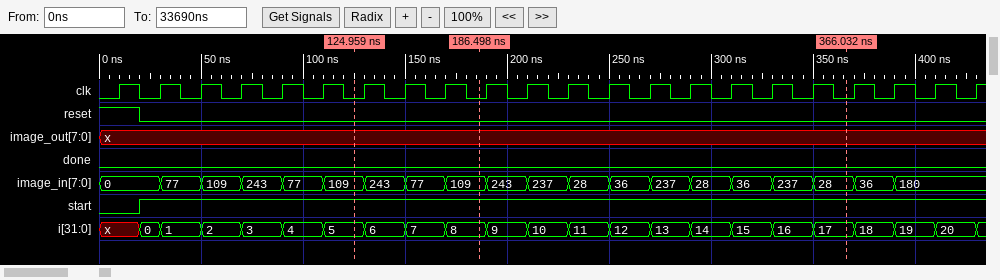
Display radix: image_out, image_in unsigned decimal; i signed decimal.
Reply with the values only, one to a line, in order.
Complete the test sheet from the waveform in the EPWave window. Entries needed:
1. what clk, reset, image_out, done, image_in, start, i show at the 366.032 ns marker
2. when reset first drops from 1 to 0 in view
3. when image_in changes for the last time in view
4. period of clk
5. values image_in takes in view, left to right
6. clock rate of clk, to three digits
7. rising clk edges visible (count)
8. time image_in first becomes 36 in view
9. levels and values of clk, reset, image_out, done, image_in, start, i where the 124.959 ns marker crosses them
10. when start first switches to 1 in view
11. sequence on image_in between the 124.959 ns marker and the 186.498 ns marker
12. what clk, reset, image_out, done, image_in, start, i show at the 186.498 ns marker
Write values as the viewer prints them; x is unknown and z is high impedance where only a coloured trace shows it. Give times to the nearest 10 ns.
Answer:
clk=0, reset=0, image_out=x, done=0, image_in=28, start=1, i=17
20 ns
390 ns
20 ns
0, 77, 109, 243, 77, 109, 243, 77, 109, 243, 237, 28, 36, 237, 28, 36, 237, 28, 36, 180
50.0 MHz
22
250 ns
clk=0, reset=0, image_out=x, done=0, image_in=109, start=1, i=5
20 ns
109, 243, 77, 109
clk=0, reset=0, image_out=x, done=0, image_in=109, start=1, i=8
